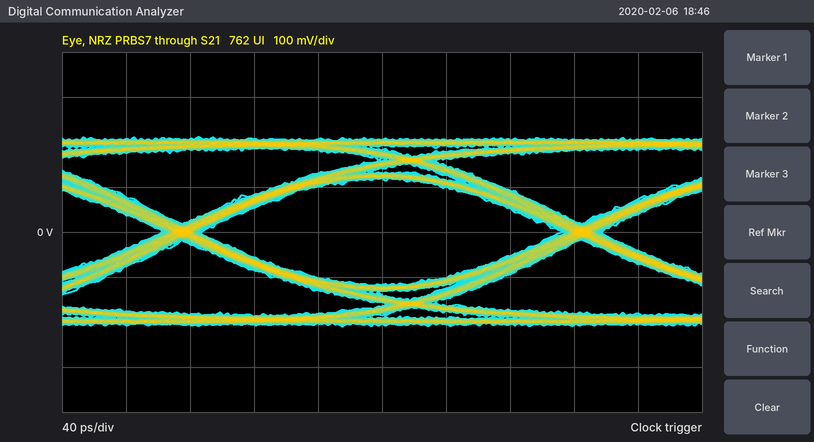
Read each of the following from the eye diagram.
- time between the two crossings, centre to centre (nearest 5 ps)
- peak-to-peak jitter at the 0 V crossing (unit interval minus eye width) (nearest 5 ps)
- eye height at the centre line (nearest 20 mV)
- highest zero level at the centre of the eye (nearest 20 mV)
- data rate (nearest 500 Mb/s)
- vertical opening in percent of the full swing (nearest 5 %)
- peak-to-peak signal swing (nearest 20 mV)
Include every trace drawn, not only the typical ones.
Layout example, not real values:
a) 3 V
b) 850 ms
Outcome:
a) 250 ps
b) 25 ps
c) 240 mV
d) -120 mV
e) 4.0 Gb/s
f) 55 %
g) 420 mV
